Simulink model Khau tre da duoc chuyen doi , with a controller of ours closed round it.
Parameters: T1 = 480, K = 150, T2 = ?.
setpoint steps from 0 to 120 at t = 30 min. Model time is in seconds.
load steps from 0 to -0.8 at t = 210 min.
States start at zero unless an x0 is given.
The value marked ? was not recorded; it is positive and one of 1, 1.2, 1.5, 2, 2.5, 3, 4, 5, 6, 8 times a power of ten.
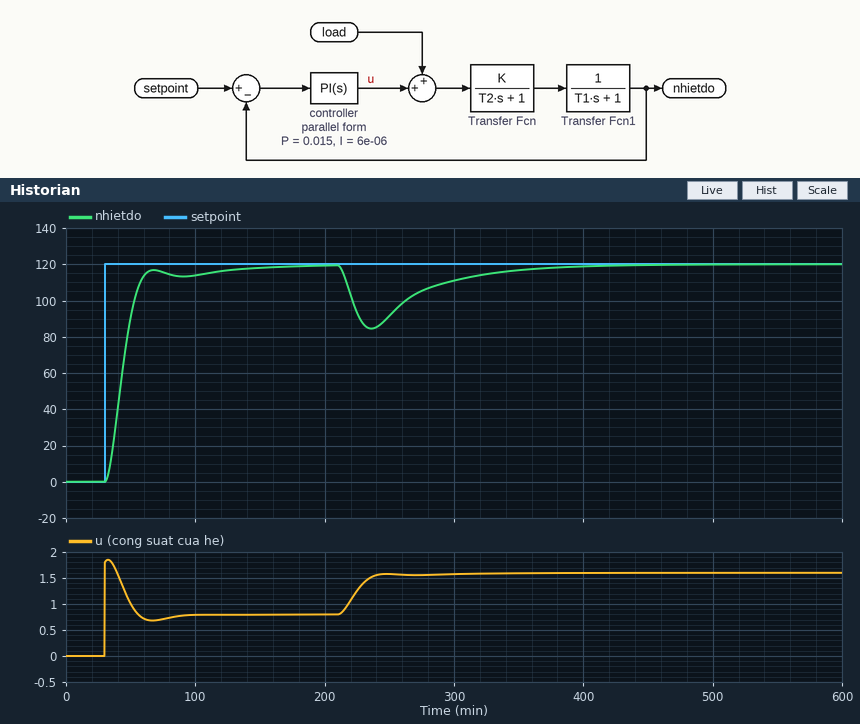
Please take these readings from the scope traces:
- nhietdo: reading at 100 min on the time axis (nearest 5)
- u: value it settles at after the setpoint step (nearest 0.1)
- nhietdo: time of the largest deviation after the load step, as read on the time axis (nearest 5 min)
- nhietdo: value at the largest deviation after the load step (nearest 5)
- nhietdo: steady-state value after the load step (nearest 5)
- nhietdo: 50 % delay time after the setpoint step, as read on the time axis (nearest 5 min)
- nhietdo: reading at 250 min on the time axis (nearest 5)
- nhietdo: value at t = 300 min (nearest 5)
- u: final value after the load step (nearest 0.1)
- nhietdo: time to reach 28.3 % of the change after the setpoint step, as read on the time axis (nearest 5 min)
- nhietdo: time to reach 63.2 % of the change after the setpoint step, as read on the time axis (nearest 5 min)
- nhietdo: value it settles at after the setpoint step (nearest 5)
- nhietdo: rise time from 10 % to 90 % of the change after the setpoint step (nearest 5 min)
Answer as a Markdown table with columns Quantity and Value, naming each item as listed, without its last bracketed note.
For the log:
| Quantity | Value |
|---|---|
| nhietdo: reading at 100 min on the time axis | 115 |
| u: value it settles at after the setpoint step | 0.8 |
| nhietdo: time of the largest deviation after the load step, as read on the time axis | 235 min |
| nhietdo: value at the largest deviation after the load step | 85 |
| nhietdo: steady-state value after the load step | 120 |
| nhietdo: 50 % delay time after the setpoint step, as read on the time axis | 45 min |
| nhietdo: reading at 250 min on the time axis | 90 |
| nhietdo: value at t = 300 min | 110 |
| u: final value after the load step | 1.6 |
| nhietdo: time to reach 28.3 % of the change after the setpoint step, as read on the time axis | 40 min |
| nhietdo: time to reach 63.2 % of the change after the setpoint step, as read on the time axis | 45 min |
| nhietdo: value it settles at after the setpoint step | 120 |
| nhietdo: rise time from 10 % to 90 % of the change after the setpoint step | 20 min |
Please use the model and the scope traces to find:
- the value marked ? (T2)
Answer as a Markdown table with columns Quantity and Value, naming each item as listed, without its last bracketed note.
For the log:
| Quantity | Value |
|---|---|
| the value marked ? | 1500 |
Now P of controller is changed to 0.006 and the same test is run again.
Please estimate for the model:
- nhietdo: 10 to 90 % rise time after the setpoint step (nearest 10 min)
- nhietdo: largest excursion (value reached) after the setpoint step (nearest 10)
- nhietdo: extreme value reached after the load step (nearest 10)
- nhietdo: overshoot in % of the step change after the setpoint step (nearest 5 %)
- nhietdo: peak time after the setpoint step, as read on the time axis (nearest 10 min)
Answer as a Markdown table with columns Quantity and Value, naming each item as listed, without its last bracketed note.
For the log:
| Quantity | Value |
|---|---|
| nhietdo: 10 to 90 % rise time after the setpoint step | 30 min |
| nhietdo: largest excursion (value reached) after the setpoint step | 130 |
| nhietdo: extreme value reached after the load step | 70 |
| nhietdo: overshoot in % of the step change after the setpoint step | 10 % |
| nhietdo: peak time after the setpoint step, as read on the time axis | 100 min |
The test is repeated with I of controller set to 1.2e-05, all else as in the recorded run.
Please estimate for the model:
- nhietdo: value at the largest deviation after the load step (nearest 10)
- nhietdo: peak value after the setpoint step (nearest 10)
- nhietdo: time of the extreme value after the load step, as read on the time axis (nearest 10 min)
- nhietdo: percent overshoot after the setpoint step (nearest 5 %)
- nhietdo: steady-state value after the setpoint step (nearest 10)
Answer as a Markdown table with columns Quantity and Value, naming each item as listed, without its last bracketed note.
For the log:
| Quantity | Value |
|---|---|
| nhietdo: value at the largest deviation after the load step | 90 |
| nhietdo: peak value after the setpoint step | 140 |
| nhietdo: time of the extreme value after the load step, as read on the time axis | 230 min |
| nhietdo: percent overshoot after the setpoint step | 15 % |
| nhietdo: steady-state value after the setpoint step | 120 |
